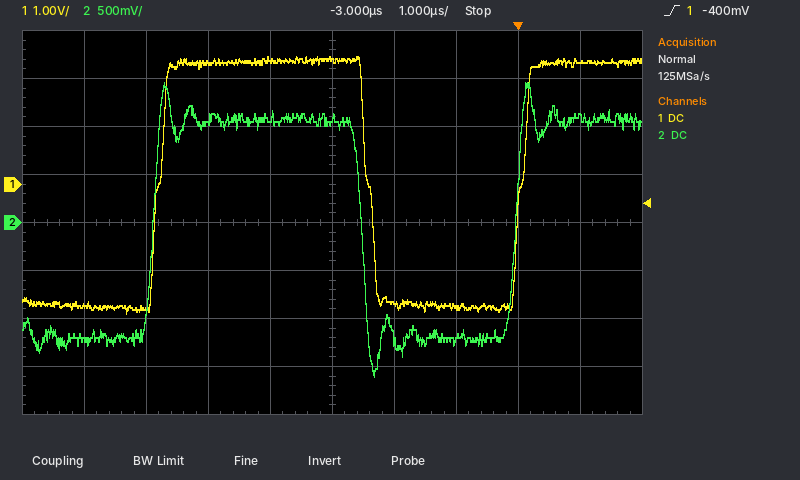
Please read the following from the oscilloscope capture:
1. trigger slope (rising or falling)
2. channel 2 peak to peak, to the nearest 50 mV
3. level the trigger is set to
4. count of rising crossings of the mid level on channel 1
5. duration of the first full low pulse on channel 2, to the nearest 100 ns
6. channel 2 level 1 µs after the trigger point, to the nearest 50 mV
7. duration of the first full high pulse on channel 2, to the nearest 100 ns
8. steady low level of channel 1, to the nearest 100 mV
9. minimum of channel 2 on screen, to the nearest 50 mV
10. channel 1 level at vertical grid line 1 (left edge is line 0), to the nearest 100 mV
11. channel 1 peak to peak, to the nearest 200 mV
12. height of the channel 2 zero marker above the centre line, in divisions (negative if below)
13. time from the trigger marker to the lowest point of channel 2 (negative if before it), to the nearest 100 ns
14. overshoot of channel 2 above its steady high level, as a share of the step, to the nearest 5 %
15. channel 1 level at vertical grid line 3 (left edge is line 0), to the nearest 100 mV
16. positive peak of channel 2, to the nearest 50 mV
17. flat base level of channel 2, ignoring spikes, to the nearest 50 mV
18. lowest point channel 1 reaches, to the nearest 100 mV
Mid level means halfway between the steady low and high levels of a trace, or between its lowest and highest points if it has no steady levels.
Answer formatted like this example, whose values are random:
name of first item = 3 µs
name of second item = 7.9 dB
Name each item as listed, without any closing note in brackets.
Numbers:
trigger slope = rising
channel 2 peak to peak, to the nearest 50 mV = 3.05 V
level the trigger is set to = -400 mV
count of rising crossings of the mid level on channel 1 = 2
duration of the first full low pulse on channel 2, to the nearest 100 ns = 2.5 µs
channel 2 level 1 µs after the trigger point, to the nearest 50 mV = 1.10 V
duration of the first full high pulse on channel 2, to the nearest 100 ns = 3.4 µs
steady low level of channel 1, to the nearest 100 mV = -2.5 V
minimum of channel 2 on screen, to the nearest 50 mV = -1.60 V
channel 1 level at vertical grid line 1 (left edge is line 0), to the nearest 100 mV = -2.5 V
channel 1 peak to peak, to the nearest 200 mV = 5.4 V
height of the channel 2 zero marker above the centre line, in divisions = 0.0 div
time from the trigger marker to the lowest point of channel 2 (negative if before it), to the nearest 100 ns = -2.3 µs
overshoot of channel 2 above its steady high level, as a share of the step, to the nearest 5 % = 15 %
channel 1 level at vertical grid line 3 (left edge is line 0), to the nearest 100 mV = 2.5 V
positive peak of channel 2, to the nearest 50 mV = 1.45 V
flat base level of channel 2, ignoring spikes, to the nearest 50 mV = -1.20 V
lowest point channel 1 reaches, to the nearest 100 mV = -2.7 V
